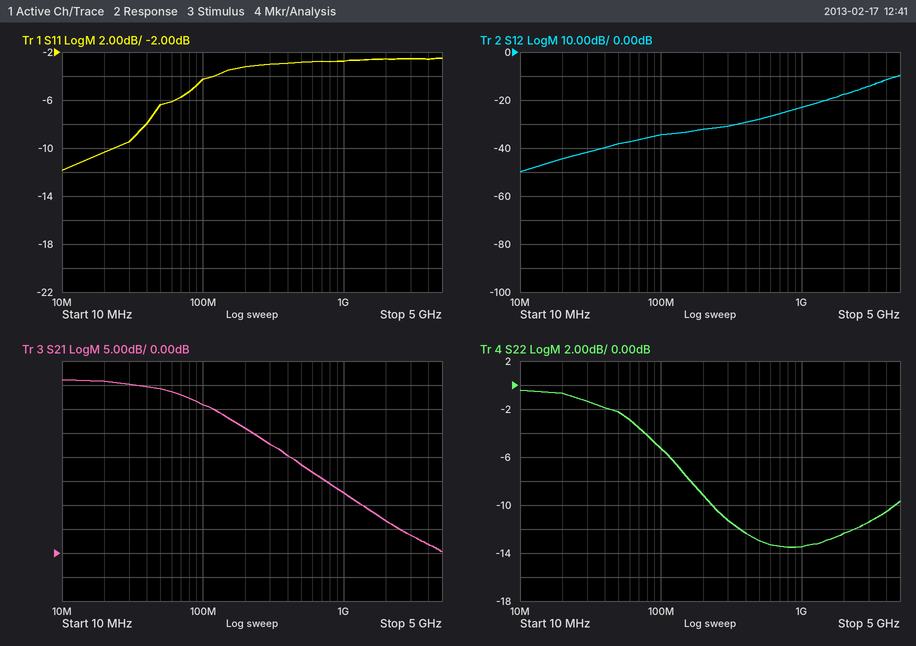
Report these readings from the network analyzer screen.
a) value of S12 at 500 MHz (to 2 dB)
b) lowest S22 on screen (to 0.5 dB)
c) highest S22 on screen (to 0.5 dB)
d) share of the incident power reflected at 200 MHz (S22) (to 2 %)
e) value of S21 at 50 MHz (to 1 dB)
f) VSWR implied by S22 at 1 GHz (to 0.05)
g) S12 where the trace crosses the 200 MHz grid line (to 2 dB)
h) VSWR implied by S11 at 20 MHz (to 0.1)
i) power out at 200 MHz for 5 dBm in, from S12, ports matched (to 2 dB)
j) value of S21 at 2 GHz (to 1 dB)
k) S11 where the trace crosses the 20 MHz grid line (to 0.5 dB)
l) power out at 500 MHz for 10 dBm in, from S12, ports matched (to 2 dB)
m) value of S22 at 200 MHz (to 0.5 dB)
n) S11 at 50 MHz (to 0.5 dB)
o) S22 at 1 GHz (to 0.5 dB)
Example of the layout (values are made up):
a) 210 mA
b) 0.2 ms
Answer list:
a) -28 dB
b) -13.5 dB
c) -0.5 dB
d) 12 %
e) 34 dB
f) 1.55
g) -32 dB
h) 1.9
i) -28 dBm
j) 7 dB
k) -10.5 dB
l) -18 dBm
m) -9.0 dB
n) -6.5 dB
o) -13.5 dB
